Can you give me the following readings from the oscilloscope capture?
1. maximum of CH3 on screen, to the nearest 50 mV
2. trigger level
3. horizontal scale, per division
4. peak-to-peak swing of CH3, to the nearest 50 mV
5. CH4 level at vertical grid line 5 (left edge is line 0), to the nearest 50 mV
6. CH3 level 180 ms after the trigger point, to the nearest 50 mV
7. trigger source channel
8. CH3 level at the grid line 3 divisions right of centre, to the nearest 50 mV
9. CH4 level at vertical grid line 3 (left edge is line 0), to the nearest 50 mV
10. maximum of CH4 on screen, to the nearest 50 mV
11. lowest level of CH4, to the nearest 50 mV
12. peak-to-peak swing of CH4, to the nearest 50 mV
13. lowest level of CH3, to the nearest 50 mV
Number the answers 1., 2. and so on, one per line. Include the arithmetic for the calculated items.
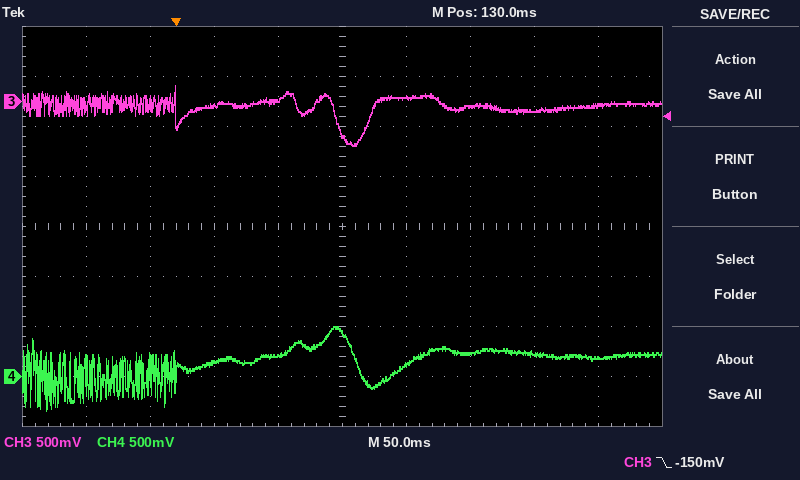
1. 150 mV
2. -150 mV
3. 50 ms
4. 150 mV − (-450 mV) = 600 mV
5. 450 mV
6. 50 mV
7. CH3
8. -100 mV
9. 150 mV
10. 500 mV
11. -350 mV
12. 500 mV − (-350 mV) = 850 mV
13. -450 mV
